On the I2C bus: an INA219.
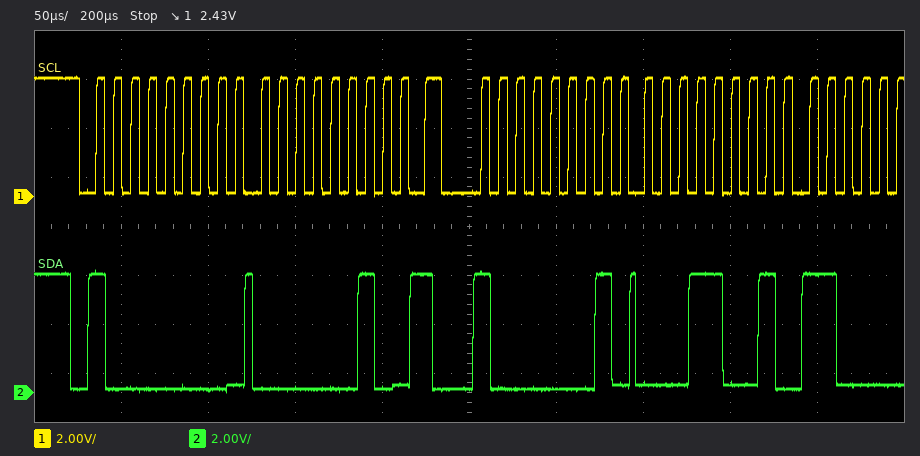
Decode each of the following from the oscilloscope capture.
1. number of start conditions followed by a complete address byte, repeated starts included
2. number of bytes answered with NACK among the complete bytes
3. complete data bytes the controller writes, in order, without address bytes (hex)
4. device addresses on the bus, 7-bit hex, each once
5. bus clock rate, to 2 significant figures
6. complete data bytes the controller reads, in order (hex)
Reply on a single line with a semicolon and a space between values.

2; 0; 02; 0x40; 100 kHz; 19
